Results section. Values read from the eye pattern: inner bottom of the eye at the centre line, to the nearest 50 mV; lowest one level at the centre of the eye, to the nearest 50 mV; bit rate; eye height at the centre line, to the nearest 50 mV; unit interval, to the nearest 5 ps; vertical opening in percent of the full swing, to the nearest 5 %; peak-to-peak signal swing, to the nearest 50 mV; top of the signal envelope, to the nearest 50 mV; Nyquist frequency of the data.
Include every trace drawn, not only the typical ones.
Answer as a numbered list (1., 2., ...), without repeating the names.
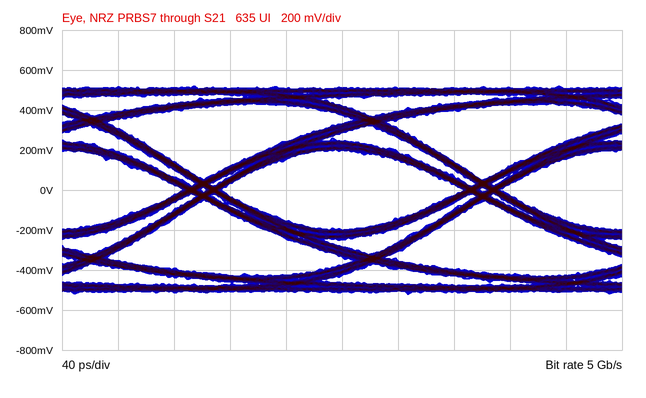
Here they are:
1. -200 mV
2. 200 mV
3. 5 Gb/s
4. 400 mV
5. 200 ps
6. 40 %
7. 1.05 V
8. 500 mV
9. 2.5 GHz
